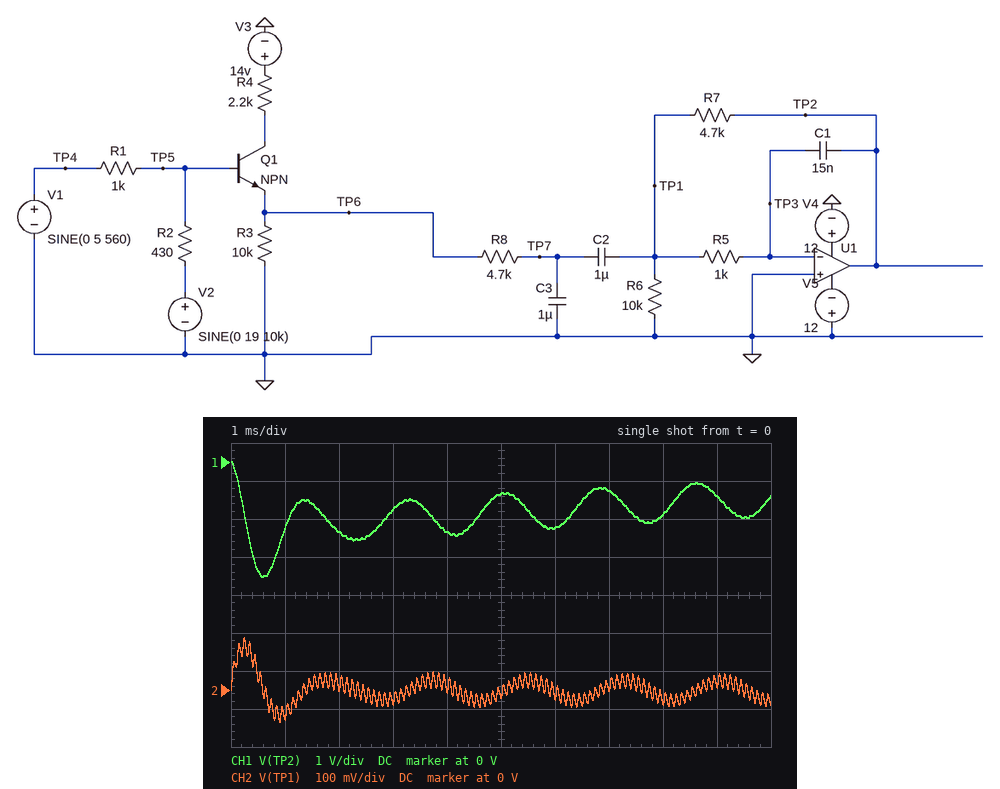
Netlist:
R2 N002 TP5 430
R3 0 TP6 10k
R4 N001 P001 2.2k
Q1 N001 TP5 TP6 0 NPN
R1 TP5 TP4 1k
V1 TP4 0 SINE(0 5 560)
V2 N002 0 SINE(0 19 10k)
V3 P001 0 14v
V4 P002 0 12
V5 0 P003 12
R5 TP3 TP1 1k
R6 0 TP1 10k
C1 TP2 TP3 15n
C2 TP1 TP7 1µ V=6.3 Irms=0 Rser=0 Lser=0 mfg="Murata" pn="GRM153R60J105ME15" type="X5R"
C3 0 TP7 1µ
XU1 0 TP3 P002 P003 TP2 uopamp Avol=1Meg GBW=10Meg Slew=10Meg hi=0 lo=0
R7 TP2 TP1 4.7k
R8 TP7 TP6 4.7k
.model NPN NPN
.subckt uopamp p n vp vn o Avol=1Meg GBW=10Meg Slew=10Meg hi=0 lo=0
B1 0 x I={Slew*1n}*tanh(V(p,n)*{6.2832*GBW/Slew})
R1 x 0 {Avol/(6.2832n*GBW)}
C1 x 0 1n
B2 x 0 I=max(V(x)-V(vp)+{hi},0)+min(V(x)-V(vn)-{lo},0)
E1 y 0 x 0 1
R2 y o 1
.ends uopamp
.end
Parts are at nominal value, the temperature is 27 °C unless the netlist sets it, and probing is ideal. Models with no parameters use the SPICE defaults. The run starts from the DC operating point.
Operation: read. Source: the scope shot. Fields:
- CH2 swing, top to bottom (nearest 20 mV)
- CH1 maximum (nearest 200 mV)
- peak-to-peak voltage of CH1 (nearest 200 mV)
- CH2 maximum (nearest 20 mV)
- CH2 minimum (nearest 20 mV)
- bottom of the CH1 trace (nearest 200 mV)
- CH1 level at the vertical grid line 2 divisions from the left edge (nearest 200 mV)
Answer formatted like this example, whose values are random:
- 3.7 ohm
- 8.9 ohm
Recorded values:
- 220 mV
- 0 V
- 3.0 V
- 140 mV
- -80 mV
- -3.0 V
- -1.8 V
